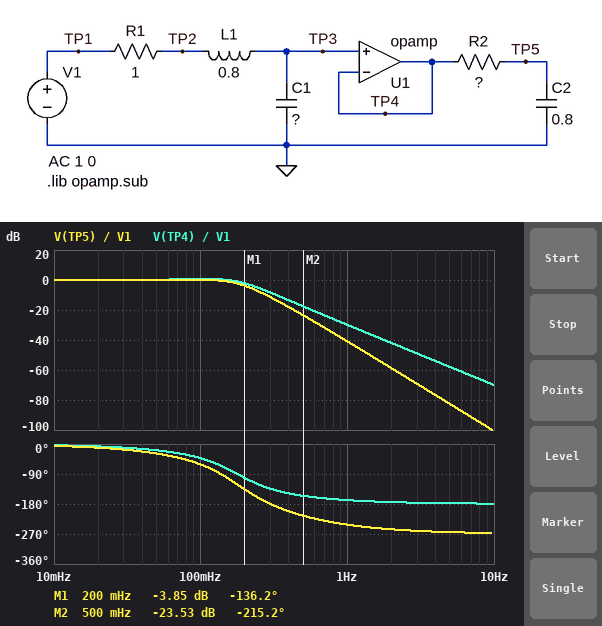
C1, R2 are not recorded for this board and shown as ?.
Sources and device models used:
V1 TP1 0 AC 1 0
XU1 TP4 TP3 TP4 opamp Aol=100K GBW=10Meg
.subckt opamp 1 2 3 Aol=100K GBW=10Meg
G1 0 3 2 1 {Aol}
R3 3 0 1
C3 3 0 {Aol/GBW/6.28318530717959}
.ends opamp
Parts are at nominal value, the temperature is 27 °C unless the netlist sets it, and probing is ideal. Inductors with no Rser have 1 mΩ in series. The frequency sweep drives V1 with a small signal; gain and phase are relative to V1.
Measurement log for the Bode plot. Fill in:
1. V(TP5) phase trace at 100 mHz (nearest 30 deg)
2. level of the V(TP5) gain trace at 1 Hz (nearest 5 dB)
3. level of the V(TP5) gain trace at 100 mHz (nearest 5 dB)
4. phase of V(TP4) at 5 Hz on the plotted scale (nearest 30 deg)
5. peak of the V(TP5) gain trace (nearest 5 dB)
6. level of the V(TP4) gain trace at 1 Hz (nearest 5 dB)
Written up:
-60 deg
-40 dB
0 dB
-180 deg
0 dB
-30 dB
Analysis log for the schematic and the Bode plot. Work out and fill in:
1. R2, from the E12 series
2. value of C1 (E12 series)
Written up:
0.68 Ω
1 F
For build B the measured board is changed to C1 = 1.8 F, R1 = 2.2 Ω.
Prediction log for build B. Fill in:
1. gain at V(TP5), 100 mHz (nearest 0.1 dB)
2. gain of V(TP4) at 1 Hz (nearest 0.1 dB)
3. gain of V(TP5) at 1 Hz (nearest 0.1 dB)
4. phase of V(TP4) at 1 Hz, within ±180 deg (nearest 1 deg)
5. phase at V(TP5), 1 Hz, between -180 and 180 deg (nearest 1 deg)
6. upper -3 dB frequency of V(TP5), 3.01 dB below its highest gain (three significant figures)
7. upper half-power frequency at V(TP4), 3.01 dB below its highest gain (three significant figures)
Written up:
-8.5 dB
-35.7 dB
-46.8 dB
-156 deg
130 deg
43.2 mHz
44.2 mHz
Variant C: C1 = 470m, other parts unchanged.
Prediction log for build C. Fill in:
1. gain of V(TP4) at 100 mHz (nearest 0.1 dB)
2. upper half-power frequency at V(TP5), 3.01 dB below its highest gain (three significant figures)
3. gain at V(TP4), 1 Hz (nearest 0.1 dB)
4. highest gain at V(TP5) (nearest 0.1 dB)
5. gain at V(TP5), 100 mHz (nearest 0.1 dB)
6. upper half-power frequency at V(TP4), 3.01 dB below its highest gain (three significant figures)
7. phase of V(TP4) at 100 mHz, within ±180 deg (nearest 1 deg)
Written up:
0.9 dB
287 mHz
-23.0 dB
1.2 dB
0.4 dB
309 mHz
-19 deg
